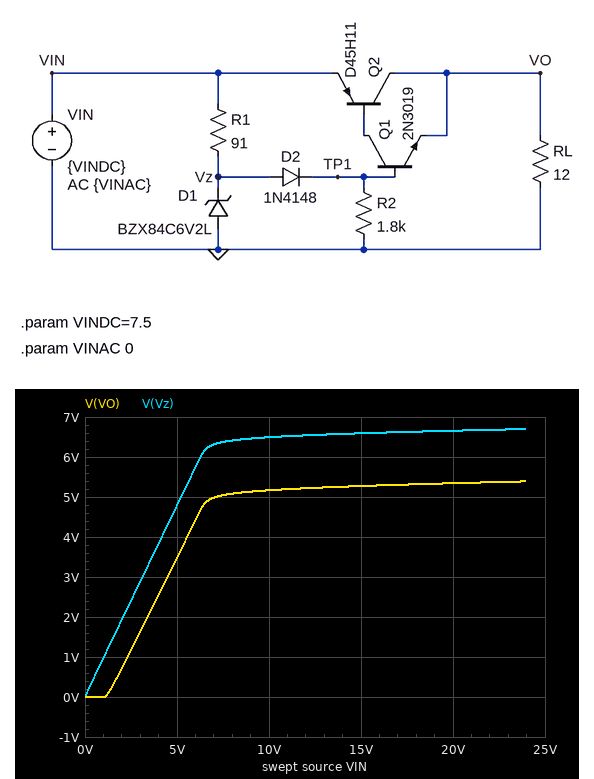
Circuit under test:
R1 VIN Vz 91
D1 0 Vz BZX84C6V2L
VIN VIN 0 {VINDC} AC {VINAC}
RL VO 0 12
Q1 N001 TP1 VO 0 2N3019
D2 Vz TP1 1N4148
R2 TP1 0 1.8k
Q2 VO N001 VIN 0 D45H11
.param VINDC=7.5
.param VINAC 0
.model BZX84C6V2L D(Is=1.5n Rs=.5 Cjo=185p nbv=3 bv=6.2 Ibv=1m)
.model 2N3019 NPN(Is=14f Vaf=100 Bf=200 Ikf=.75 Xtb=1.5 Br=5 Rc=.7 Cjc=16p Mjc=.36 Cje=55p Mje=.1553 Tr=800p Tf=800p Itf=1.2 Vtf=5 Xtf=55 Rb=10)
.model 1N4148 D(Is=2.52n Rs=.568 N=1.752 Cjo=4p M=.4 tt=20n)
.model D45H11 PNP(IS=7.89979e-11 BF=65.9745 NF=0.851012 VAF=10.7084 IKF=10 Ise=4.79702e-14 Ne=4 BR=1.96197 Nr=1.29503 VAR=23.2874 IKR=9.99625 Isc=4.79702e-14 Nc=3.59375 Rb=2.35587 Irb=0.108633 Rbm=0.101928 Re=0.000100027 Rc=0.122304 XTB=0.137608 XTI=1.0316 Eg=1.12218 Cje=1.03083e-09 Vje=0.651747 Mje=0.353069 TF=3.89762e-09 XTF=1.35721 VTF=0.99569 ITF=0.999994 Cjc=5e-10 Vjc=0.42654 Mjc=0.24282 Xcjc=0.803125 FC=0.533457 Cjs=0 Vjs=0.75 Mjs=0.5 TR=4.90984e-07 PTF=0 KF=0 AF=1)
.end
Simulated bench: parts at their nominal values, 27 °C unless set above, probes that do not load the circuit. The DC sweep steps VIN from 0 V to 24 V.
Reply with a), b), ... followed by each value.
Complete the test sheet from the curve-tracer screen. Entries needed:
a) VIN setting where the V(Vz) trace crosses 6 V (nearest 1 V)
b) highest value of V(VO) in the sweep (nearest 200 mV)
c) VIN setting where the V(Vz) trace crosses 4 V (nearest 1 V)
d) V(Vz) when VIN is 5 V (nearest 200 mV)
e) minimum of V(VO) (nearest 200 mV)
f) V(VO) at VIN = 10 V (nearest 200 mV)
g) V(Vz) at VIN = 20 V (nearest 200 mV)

a) 6 V
b) 5.4 V
c) 4 V
d) 4.8 V
e) 0 V
f) 5.2 V
g) 6.6 V
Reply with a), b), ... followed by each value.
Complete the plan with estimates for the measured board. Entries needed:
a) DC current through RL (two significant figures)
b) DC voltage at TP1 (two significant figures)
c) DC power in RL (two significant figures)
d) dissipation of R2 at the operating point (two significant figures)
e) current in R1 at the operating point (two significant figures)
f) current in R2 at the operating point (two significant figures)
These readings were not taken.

a) 420 mA
b) 5.7 V
c) 2.1 W
d) 18 mW
e) 12 mA
f) 3.2 mA
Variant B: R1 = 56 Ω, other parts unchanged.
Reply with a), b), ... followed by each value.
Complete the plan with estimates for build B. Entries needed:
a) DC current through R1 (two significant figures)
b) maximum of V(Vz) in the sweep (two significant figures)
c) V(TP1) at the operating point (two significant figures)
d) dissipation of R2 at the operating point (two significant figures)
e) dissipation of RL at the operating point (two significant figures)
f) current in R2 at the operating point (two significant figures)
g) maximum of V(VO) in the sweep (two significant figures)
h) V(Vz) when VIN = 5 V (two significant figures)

a) 19 mA
b) 6.8 V
c) 5.8 V
d) 19 mW
e) 2.2 W
f) 3.2 mA
g) 5.5 V
h) 4.9 V
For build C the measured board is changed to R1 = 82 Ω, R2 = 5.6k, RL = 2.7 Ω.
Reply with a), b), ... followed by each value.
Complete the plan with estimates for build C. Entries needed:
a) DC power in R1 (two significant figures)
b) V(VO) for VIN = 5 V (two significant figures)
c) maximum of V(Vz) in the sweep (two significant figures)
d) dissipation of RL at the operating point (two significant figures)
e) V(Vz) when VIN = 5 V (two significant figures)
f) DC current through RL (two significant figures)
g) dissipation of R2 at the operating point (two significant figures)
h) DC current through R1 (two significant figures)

a) 15 mW
b) 3.6 V
c) 6.7 V
d) 9.5 W
e) 4.9 V
f) 1.9 A
g) 6.0 mW
h) 13 mA
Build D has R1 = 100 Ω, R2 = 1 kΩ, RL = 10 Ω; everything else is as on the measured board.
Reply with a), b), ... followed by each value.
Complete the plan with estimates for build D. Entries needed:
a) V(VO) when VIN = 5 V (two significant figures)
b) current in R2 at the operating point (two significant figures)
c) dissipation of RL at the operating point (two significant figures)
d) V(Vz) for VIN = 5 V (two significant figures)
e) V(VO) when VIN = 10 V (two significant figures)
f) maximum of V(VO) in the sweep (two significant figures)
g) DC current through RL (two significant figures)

a) 3.3 V
b) 5.7 mA
c) 2.5 W
d) 4.6 V
e) 5.1 V
f) 5.3 V
g) 500 mA
